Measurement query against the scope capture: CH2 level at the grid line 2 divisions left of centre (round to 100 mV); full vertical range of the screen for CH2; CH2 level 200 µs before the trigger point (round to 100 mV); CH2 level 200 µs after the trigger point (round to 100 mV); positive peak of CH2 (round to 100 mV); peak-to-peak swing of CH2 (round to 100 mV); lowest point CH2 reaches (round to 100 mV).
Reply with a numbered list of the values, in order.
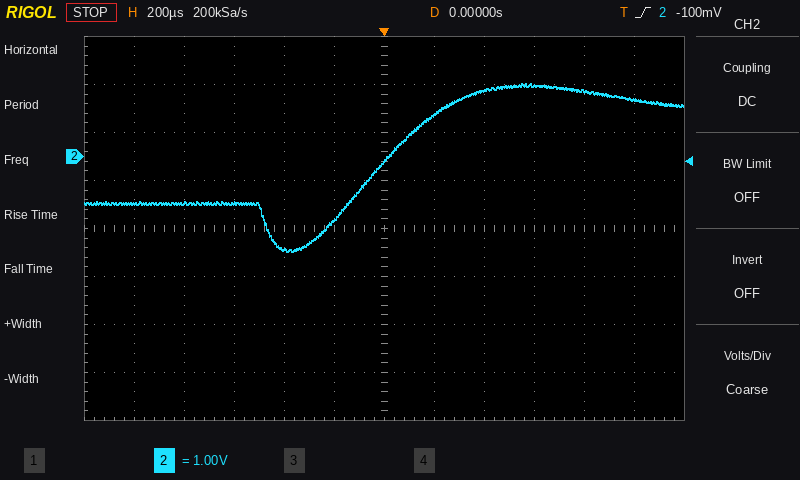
1. -1.9 V
2. 8 V
3. -1.3 V
4. 900 mV
5. 1.5 V
6. 3.5 V
7. -2.0 V
